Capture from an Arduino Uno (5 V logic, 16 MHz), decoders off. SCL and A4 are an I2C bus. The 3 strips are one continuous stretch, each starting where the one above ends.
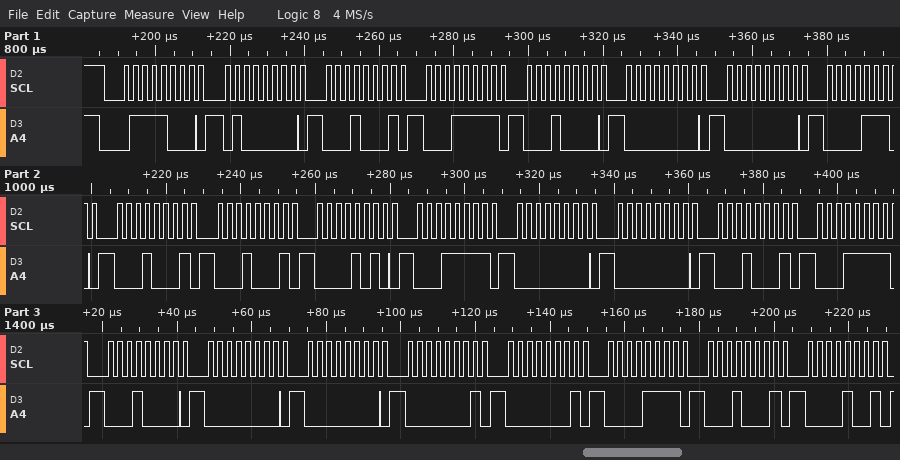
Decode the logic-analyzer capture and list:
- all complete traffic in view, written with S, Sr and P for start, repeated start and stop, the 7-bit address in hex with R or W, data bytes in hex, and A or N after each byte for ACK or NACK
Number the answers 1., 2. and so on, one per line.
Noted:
1. S 3CW A 40 A 11 A 1F A 10 A 00 A 00 A 0E A 11 A 11 A 0A A 1F A 00 A 00 A 11 A 1F A 10 A 00 A 00 A 01 A 01 A 0F A 11 A 09 A
